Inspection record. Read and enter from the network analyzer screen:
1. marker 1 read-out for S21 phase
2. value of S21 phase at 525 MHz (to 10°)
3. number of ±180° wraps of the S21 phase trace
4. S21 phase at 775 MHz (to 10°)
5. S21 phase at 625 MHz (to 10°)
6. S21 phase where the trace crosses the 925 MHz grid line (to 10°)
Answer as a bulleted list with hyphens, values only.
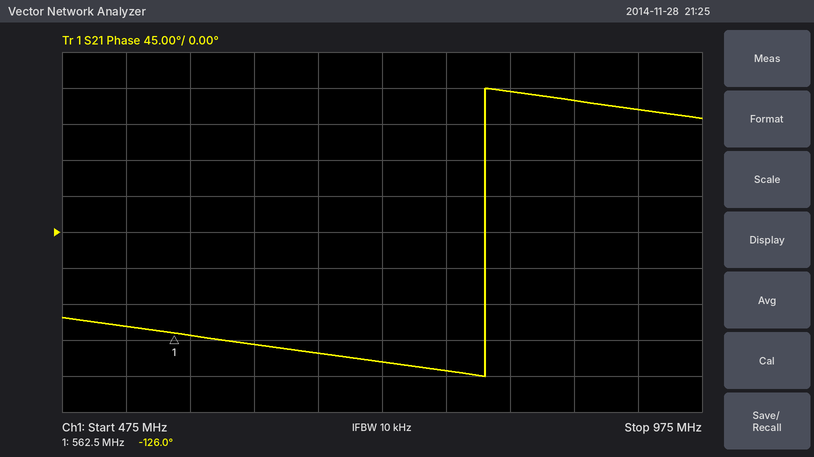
- -126.0°
- -120°
- 1
- -170°
- -140°
- 150°
